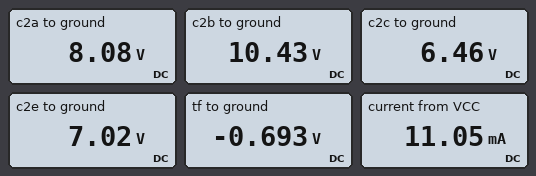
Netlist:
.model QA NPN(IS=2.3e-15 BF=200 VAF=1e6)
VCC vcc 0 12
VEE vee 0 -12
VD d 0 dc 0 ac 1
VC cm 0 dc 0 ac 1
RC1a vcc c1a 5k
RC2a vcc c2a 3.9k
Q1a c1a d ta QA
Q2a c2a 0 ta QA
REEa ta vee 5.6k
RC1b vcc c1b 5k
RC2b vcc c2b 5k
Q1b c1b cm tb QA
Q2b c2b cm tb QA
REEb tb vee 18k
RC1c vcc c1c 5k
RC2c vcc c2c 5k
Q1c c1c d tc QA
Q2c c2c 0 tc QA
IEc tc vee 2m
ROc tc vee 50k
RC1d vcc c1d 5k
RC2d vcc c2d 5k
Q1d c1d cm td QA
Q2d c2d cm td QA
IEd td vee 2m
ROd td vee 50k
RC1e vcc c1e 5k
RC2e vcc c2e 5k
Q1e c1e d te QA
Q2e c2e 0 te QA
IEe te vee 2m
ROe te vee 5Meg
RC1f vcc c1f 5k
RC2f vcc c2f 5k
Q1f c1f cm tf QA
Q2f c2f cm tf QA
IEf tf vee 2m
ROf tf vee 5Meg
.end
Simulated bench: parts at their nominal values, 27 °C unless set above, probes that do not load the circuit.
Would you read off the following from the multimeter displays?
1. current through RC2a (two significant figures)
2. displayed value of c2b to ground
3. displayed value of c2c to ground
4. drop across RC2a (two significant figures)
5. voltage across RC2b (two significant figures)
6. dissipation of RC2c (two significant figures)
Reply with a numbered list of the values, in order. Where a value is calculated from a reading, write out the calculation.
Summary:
1. (12 V - 8.08 V) / 3.9 kΩ = 1.0 mA
2. 10.43 V
3. 6.46 V
4. 12 V - 8.08 V = 3.9 V
5. 12 V - 10.43 V = 1.6 V
6. (12 V - 6.46 V)^2 / 5 kΩ = 6.1 mW
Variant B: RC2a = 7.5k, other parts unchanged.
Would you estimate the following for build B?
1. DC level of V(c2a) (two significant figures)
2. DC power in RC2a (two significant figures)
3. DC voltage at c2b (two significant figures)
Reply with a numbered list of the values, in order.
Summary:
1. 4.5 V
2. 7.6 mW
3. 10 V
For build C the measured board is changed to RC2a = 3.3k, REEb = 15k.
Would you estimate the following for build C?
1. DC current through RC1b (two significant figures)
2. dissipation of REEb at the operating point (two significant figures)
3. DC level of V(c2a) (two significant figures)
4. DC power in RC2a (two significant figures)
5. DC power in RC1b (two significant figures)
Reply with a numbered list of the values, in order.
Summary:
1. 380 µA
2. 8.6 mW
3. 8.7 V
4. 3.3 mW
5. 710 µW
